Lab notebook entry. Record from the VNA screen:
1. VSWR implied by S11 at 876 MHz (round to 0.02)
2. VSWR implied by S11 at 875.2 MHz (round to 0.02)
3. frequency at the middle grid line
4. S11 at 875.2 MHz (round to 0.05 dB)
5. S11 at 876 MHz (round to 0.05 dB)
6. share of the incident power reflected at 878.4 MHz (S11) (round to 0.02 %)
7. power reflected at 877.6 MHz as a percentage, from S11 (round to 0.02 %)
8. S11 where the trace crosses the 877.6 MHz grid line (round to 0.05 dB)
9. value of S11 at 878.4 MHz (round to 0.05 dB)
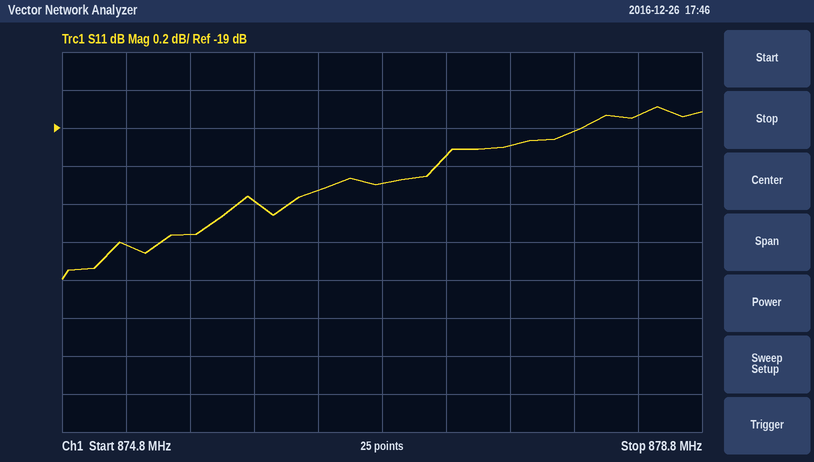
1.24
1.24
876.8 MHz
-19.60 dB
-19.40 dB
1.28 %
1.24 %
-19.10 dB
-18.95 dB
